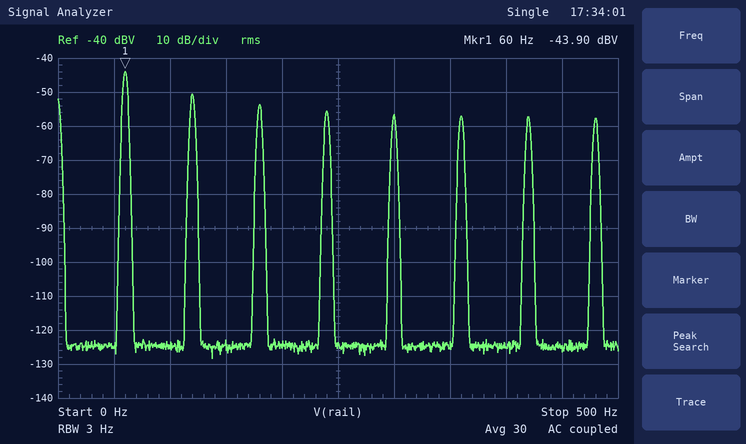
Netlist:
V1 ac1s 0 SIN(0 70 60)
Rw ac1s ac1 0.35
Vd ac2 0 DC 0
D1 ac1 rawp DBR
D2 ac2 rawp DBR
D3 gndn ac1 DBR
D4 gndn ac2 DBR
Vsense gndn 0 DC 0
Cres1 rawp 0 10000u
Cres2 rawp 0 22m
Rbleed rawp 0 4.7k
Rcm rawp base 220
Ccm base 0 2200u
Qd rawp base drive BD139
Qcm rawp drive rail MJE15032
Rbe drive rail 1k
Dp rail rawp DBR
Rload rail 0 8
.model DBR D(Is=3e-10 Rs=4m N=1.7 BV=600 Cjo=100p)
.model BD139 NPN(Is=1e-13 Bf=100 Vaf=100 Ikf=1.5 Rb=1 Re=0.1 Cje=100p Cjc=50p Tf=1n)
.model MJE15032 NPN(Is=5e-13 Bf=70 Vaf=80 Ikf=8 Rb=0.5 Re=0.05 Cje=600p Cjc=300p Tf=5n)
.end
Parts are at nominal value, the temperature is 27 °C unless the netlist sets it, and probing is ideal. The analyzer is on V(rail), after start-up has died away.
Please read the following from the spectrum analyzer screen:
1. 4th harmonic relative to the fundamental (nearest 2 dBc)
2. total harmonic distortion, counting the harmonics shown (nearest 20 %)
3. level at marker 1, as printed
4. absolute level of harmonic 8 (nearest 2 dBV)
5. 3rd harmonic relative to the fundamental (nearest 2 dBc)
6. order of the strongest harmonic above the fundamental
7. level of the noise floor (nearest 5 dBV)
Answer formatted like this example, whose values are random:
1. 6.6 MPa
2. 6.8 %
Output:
1. -12 dBc
2. 80 %
3. -43.90 dBV
4. -58 dBV
5. -10 dBc
6. 2
7. -125 dBV
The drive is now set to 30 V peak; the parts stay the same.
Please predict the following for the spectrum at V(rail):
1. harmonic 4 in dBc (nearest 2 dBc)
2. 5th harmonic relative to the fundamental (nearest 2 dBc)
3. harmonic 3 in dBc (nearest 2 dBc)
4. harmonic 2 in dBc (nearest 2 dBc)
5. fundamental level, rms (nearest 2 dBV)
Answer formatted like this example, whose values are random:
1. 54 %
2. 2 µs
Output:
1. -28 dBc
2. -36 dBc
3. -20 dBc
4. -12 dBc
5. -56 dBV
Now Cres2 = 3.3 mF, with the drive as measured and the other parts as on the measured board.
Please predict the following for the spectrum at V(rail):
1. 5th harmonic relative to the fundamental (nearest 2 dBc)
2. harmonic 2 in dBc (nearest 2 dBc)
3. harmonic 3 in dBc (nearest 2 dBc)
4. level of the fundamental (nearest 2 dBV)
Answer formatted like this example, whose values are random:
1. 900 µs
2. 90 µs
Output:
1. -8 dBc
2. -4 dBc
3. -6 dBc
4. -32 dBV
